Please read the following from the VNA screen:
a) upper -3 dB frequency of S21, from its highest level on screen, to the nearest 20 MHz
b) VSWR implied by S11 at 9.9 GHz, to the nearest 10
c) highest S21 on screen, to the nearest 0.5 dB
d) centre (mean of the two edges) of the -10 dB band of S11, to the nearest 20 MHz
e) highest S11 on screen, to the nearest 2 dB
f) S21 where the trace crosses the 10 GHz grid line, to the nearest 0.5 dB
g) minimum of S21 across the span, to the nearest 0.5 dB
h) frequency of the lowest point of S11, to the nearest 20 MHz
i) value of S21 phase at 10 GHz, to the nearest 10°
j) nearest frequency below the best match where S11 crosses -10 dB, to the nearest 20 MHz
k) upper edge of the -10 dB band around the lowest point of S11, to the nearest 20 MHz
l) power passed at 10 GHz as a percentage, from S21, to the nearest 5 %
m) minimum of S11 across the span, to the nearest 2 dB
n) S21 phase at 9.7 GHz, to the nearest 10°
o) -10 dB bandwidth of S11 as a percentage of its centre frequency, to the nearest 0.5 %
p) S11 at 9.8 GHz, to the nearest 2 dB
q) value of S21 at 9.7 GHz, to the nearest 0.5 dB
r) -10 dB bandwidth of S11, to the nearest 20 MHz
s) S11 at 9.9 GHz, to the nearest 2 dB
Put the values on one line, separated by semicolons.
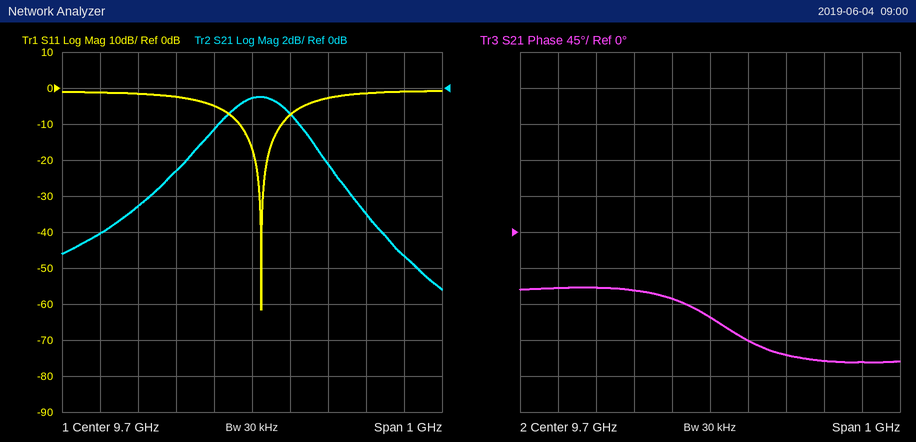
9.88 GHz; 10; -0.5 dB; 9.72 GHz; 0 dB; -7.0 dB; -11.0 dB; 9.72 GHz; -160°; 9.66 GHz; 9.78 GHz; 20 %; -62 dB; -110°; 1.0 %; -8 dB; -0.5 dB; 120 MHz; -2 dB
